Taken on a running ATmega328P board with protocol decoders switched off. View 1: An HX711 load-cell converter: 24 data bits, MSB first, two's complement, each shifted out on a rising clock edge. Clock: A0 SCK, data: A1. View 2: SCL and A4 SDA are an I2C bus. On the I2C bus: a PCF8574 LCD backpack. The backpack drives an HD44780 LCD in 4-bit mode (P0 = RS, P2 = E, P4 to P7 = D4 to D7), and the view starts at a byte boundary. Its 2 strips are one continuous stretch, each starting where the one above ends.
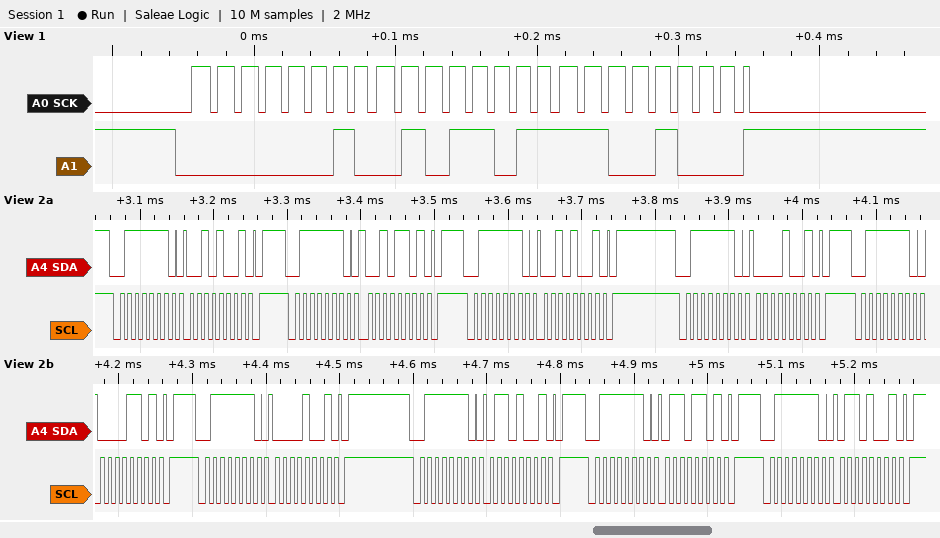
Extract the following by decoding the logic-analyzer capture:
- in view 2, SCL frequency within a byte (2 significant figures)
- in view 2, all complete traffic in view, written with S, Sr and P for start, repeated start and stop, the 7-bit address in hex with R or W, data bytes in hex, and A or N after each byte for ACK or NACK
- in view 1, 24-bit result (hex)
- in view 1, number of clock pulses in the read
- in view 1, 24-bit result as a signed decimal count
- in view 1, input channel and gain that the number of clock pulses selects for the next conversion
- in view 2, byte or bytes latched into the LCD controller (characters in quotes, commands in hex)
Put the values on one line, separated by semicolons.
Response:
100 kHz; S 3FW A 29 A P S 3FW A 2D A P S 3FW A 29 A P S 3FW A 09 A P S 3FW A 0D A P S 3FW A 09 A P S 3FW A 69 A P S 3FW A 6D A P S 3FW A 69 A P; 0x025BC8; 25; 154568; channel A, gain 128; ' '
